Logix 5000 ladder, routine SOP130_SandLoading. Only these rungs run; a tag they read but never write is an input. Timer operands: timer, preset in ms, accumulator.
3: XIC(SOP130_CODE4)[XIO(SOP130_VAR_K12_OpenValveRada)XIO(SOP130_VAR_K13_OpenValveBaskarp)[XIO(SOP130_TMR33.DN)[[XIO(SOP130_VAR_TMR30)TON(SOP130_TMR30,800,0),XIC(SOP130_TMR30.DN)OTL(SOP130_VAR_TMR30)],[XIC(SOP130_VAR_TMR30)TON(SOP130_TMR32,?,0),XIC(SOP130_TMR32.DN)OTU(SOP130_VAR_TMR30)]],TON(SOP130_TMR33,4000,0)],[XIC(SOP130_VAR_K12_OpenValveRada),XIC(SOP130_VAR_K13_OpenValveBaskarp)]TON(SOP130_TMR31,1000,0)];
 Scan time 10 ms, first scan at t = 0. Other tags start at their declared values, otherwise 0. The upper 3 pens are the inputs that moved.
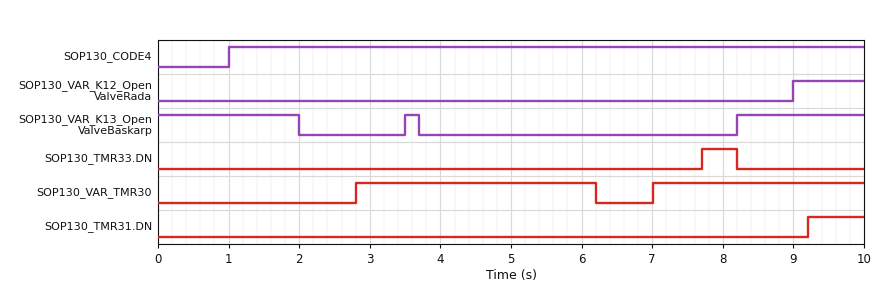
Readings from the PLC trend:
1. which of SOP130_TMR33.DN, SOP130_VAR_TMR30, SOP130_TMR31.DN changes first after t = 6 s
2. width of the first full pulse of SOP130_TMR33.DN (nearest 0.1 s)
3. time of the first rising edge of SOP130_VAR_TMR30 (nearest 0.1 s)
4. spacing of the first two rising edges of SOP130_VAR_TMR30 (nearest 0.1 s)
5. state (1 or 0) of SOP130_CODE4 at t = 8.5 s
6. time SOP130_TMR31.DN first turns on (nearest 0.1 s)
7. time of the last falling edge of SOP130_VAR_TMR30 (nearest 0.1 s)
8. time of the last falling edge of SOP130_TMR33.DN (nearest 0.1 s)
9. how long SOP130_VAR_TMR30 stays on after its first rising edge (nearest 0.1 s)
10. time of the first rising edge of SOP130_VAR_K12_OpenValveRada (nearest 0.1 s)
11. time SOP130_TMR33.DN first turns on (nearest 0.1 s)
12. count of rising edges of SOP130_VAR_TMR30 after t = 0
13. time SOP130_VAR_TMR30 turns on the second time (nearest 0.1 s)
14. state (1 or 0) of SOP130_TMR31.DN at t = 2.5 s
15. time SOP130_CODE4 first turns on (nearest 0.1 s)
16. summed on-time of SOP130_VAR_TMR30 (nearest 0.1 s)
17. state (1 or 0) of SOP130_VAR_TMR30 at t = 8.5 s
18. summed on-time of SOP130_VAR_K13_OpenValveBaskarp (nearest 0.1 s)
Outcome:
SOP130_VAR_TMR30
0.5 s
2.8 s
4.2 s
1
9.2 s
6.2 s
8.2 s
3.4 s
9.0 s
7.7 s
2
7.0 s
0
1.0 s
6.4 s
1
4.0 s
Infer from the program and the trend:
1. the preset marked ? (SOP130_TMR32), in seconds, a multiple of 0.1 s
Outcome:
2.5 s
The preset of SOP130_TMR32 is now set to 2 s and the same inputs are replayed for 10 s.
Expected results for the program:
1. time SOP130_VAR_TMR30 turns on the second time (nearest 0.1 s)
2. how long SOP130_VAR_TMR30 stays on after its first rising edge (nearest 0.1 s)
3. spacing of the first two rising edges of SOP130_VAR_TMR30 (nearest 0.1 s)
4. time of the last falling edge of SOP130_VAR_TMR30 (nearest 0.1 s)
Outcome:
6.5 s
2.9 s
3.7 s
5.7 s
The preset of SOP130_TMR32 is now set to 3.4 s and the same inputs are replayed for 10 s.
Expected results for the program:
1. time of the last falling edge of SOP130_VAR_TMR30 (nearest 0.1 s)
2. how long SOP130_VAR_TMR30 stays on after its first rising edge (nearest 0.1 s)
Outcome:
7.1 s
4.3 s
